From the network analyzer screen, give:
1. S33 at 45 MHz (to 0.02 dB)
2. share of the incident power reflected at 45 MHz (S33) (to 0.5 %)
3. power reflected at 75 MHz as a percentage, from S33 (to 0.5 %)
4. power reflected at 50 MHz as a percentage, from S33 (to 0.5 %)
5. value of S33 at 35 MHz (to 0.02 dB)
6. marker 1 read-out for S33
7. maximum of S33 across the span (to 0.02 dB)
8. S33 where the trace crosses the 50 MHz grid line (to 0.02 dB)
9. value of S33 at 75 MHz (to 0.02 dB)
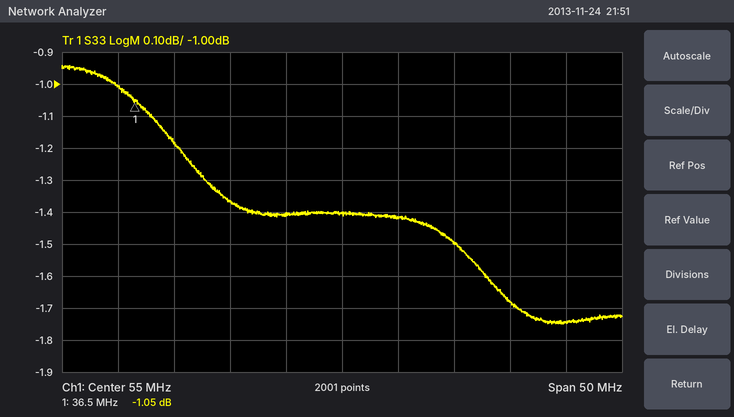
-1.36 dB
73.0 %
67.0 %
72.5 %
-1.00 dB
-1.05 dB
-0.94 dB
-1.40 dB
-1.74 dB
